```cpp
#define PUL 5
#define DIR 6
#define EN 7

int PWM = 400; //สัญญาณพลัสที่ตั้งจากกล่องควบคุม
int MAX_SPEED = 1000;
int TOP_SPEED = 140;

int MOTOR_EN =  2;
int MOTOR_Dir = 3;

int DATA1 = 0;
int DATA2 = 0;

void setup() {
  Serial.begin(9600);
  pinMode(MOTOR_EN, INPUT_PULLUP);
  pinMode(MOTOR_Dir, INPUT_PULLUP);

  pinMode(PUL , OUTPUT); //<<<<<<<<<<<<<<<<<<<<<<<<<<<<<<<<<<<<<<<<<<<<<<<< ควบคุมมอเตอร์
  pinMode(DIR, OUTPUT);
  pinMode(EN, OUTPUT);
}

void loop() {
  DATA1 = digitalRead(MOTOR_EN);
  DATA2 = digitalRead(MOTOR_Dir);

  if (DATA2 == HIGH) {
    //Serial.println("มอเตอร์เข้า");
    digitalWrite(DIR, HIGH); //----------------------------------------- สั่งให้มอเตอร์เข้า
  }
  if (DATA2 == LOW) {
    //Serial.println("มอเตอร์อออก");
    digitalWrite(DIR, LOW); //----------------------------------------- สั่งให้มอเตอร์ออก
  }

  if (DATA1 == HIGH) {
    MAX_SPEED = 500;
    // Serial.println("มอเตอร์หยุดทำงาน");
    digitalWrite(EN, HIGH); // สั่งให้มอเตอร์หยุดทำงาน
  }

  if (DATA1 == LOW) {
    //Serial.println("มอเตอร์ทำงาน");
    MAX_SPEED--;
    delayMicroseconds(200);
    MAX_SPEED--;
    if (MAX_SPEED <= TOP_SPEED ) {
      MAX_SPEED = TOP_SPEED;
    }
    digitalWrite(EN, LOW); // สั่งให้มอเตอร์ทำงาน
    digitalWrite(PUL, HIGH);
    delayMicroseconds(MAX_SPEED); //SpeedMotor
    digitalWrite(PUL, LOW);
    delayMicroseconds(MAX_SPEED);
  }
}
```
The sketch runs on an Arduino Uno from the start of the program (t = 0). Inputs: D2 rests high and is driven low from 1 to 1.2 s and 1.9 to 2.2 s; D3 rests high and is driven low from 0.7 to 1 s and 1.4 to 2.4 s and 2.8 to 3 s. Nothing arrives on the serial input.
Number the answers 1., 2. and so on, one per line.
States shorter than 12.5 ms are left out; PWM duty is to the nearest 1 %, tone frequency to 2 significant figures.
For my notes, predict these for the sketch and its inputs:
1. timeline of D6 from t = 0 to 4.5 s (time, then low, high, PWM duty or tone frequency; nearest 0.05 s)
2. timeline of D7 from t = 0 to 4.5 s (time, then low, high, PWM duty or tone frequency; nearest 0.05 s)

1. 0 s high; 0.7 s low; 1 s high; 1.4 s low; 2.4 s high; 2.8 s low; 3 s high
2. 0 s high; 1 s low; 1.2 s high; 1.9 s low; 2.2 s high
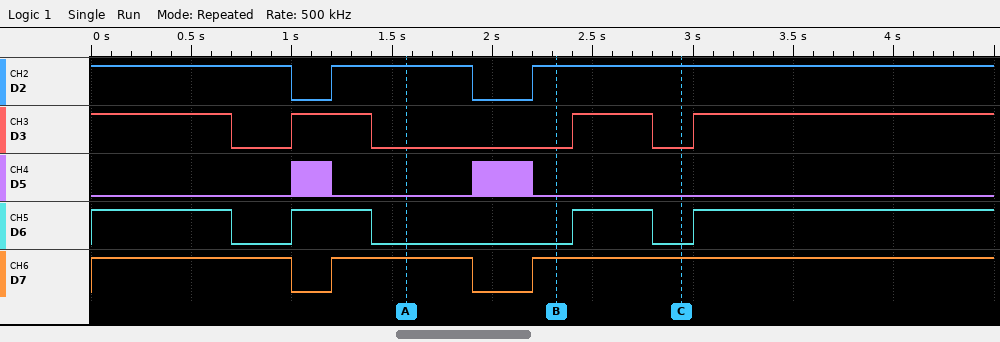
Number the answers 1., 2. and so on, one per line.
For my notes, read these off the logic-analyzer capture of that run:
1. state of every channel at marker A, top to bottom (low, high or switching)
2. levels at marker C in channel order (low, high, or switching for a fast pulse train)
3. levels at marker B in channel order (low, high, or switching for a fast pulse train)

1. D2 high, D3 low, D5 low, D6 low, D7 high
2. D2 high, D3 low, D5 low, D6 low, D7 high
3. D2 high, D3 low, D5 low, D6 low, D7 high
